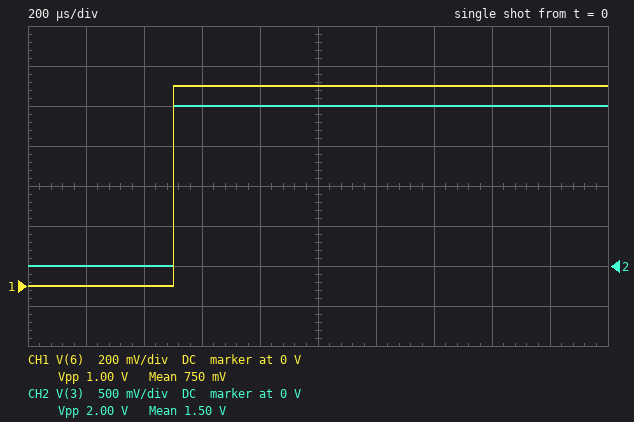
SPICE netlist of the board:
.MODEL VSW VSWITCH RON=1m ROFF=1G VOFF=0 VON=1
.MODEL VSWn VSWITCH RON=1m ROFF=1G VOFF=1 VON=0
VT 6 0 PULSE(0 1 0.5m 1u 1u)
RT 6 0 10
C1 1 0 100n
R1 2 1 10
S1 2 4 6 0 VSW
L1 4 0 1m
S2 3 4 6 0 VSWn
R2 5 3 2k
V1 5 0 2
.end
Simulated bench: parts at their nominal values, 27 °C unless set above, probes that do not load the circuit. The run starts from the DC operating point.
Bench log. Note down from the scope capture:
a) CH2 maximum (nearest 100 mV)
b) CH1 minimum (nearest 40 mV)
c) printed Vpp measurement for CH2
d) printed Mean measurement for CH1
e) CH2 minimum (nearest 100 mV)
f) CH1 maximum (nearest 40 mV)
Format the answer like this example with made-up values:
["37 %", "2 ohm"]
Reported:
["2.0 V", "0 V", "2.00 V", "750 mV", "0 V", "1.00 V"]
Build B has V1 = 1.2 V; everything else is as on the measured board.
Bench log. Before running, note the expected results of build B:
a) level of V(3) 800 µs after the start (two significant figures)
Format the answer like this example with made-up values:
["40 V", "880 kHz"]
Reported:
["1.2 V"]
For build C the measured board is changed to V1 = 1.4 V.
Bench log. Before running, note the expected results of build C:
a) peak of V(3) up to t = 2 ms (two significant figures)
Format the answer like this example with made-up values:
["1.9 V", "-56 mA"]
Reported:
["1.4 V"]
